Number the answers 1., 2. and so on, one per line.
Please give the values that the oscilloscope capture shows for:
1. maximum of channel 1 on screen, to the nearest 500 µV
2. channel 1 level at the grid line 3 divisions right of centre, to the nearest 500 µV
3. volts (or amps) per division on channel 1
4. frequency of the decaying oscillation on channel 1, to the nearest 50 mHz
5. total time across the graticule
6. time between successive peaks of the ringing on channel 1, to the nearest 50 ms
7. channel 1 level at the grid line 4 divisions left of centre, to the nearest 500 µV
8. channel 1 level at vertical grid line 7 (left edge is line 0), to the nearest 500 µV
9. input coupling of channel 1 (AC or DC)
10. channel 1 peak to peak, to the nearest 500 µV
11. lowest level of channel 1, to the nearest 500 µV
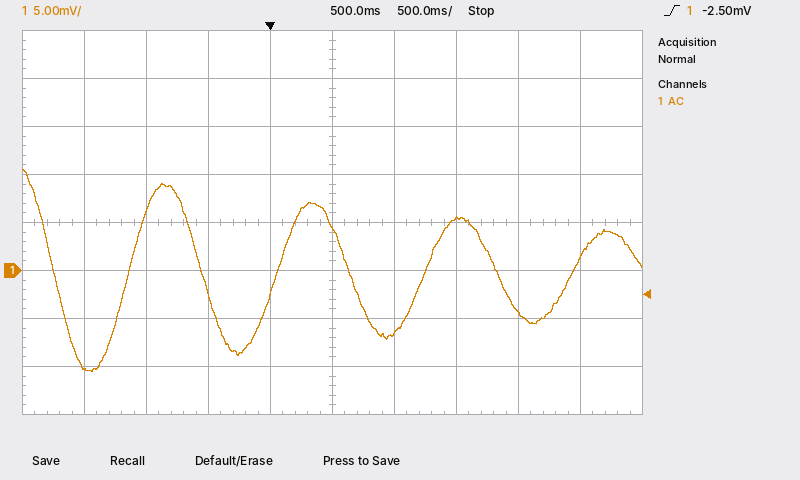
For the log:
1. 10.5 mV
2. -4.5 mV
3. 5 mV
4. 850 mHz
5. 5 s
6. 1.20 s
7. -10.0 mV
8. 5.5 mV
9. AC
10. 21.0 mV
11. -10.5 mV
